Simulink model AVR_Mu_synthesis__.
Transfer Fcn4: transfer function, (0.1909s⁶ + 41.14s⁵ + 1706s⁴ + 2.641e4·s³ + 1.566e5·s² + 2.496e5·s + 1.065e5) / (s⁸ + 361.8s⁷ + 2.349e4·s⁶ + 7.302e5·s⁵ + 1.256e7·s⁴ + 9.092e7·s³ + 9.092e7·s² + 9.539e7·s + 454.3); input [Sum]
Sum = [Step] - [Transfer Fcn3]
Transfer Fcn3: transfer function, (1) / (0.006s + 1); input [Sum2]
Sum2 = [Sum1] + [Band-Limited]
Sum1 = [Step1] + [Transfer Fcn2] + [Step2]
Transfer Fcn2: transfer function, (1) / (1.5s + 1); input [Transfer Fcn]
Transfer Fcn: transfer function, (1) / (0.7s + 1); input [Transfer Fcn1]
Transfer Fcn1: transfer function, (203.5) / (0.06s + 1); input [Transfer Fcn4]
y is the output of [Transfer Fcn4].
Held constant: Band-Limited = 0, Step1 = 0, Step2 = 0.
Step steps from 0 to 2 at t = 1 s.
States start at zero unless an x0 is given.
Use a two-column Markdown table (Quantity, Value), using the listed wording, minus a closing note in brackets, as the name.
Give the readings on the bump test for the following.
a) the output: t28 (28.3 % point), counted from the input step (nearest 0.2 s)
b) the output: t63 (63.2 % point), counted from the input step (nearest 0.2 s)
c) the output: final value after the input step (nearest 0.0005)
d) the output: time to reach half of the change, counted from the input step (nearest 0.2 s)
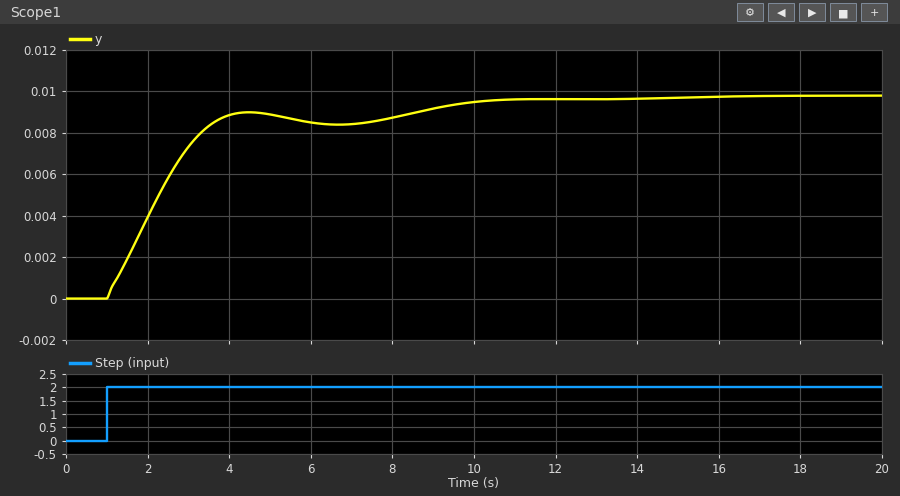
| Quantity | Value |
|---|---|
| the output: t28 (28.3 % point), counted from the input step | 0.8 s |
| the output: t63 (63.2 % point), counted from the input step | 1.6 s |
| the output: final value after the input step | 0.0100 |
| the output: time to reach half of the change, counted from the input step | 1.2 s |
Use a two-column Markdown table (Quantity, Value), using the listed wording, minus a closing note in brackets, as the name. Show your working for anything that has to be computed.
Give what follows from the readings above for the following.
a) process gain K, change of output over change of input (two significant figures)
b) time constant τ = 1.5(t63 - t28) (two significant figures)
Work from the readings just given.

| Quantity | Value |
|---|---|
| process gain K, change of output over change of input | (0.01 - 0) / 2 = 0.0050 |
| time constant τ = 1.5(t63 - t28) | 1.5 × (1.6 - 0.8) = 1.2 s |
